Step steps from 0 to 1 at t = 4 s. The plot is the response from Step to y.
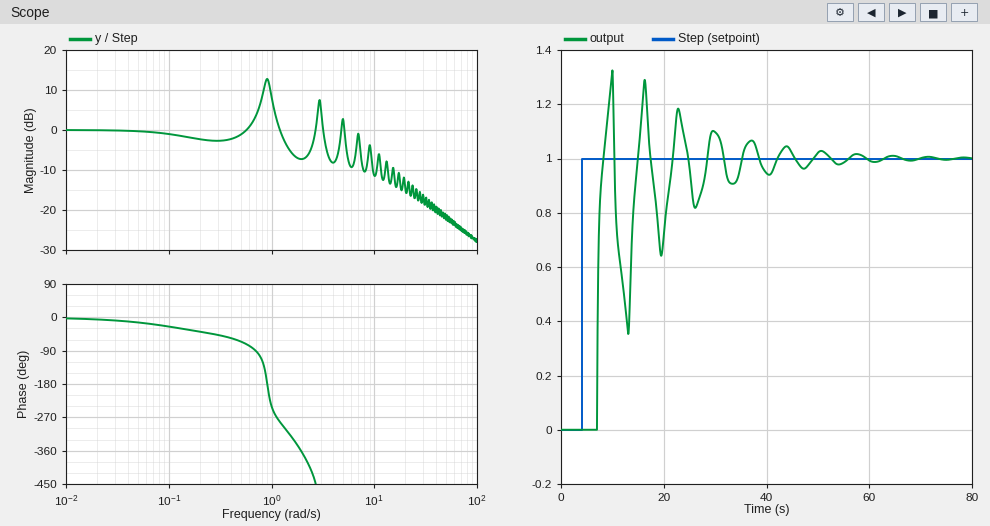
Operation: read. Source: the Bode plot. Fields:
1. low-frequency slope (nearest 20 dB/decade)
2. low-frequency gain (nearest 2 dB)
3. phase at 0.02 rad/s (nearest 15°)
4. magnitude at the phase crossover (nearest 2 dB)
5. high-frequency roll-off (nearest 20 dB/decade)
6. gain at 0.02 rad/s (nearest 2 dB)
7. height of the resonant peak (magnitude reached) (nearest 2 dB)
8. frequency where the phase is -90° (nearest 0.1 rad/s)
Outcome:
0 dB/decade
0 dB
0°
12 dB
-20 dB/decade
0 dB
12 dB
0.7 rad/s
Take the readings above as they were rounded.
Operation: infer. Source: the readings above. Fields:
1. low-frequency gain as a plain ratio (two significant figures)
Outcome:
1.0
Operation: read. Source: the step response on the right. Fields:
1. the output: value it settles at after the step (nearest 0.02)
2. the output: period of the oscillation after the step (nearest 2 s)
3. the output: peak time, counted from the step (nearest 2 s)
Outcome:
1.00
6 s
6 s
